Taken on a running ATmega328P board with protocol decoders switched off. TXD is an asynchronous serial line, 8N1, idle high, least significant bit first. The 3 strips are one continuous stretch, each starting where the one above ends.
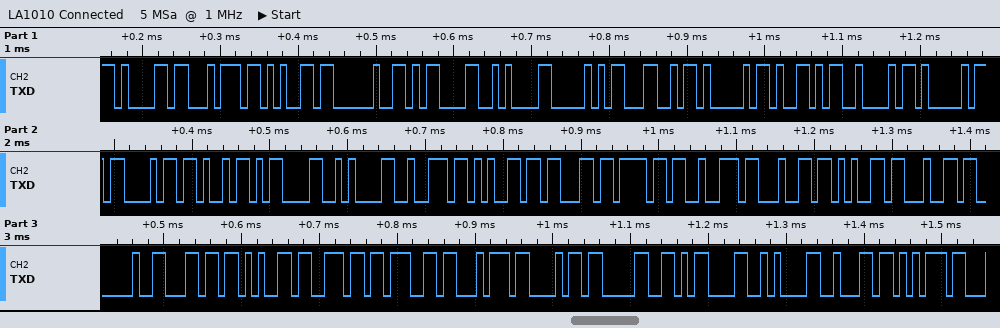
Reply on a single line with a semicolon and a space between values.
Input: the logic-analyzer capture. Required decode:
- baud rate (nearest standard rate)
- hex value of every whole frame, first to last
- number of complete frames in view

115200 baud; 61 74 65 20 0D 0A 50 4C 41 59 42 41 43 4B 0D 0A 72 65 63 6F 72 64 65 64 20 6C 65 6E 67 74 68 30 0D 0A 62 75; 36
